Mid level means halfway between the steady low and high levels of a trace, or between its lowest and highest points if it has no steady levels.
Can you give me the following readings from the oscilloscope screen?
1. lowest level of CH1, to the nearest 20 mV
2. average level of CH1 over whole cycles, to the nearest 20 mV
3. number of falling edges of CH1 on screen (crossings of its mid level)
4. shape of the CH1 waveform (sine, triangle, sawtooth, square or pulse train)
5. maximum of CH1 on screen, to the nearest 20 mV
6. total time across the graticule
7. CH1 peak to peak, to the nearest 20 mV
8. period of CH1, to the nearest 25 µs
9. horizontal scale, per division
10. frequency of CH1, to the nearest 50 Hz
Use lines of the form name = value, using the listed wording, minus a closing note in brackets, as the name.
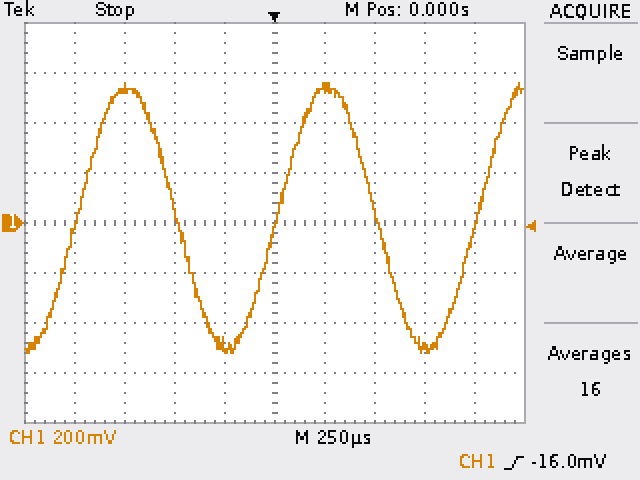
lowest level of CH1, to the nearest 20 mV = -520 mV
average level of CH1 over whole cycles, to the nearest 20 mV = 20 mV
number of falling edges of CH1 on screen = 2
shape of the CH1 waveform = sine
maximum of CH1 on screen, to the nearest 20 mV = 560 mV
total time across the graticule = 2.5 ms
CH1 peak to peak, to the nearest 20 mV = 1.08 V
period of CH1, to the nearest 25 µs = 1.000 ms
horizontal scale, per division = 250 µs
frequency of CH1, to the nearest 50 Hz = 1.00 kHz
